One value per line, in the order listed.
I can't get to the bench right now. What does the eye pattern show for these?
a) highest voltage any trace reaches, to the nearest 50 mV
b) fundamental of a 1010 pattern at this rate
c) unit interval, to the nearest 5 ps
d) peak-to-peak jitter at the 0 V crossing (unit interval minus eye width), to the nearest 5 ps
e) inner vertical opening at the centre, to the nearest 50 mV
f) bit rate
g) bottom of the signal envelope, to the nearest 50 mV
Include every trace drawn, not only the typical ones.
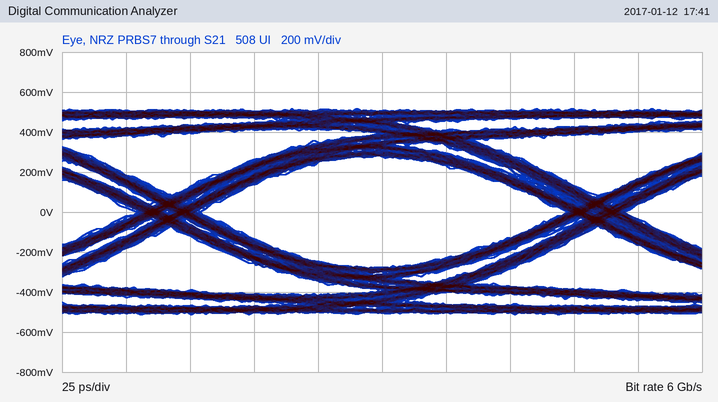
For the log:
500 mV
3 GHz
165 ps
25 ps
550 mV
6 Gb/s
-500 mV
